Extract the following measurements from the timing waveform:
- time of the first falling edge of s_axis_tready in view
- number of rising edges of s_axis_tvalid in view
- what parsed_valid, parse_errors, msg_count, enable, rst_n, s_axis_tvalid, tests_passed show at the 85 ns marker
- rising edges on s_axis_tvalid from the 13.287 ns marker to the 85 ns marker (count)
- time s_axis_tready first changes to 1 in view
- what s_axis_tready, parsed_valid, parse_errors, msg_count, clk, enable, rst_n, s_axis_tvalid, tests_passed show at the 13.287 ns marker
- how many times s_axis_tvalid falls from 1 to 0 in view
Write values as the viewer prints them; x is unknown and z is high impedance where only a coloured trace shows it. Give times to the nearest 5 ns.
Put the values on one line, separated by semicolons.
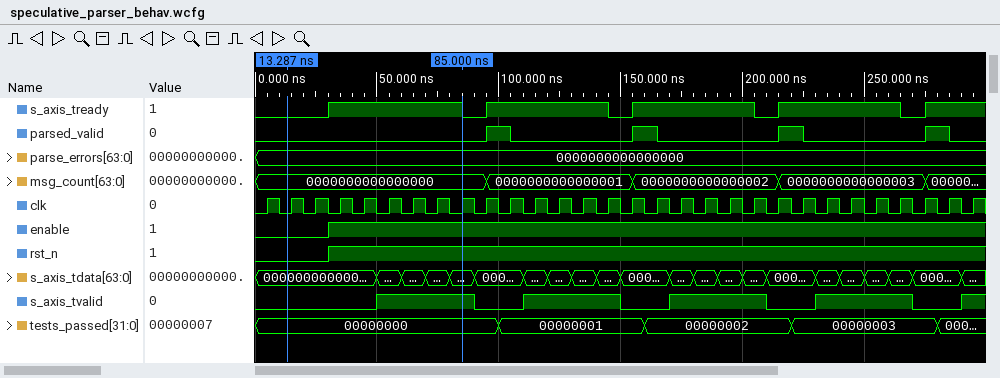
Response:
85 ns; 5; parsed_valid=0, parse_errors=0000000000000000, msg_count=0000000000000000, enable=1, rst_n=1, s_axis_tvalid=1, tests_passed=00000000; 1; 30 ns; s_axis_tready=0, parsed_valid=0, parse_errors=0000000000000000, msg_count=0000000000000000, clk=0, enable=0, rst_n=0, s_axis_tvalid=0, tests_passed=00000000; 4
